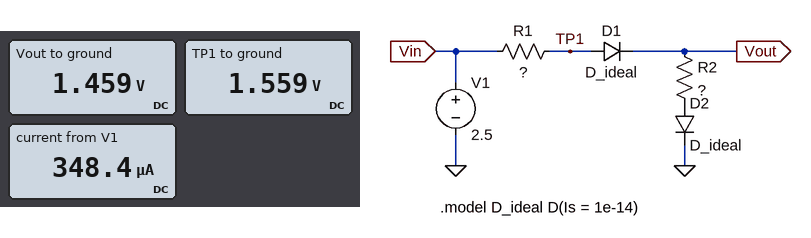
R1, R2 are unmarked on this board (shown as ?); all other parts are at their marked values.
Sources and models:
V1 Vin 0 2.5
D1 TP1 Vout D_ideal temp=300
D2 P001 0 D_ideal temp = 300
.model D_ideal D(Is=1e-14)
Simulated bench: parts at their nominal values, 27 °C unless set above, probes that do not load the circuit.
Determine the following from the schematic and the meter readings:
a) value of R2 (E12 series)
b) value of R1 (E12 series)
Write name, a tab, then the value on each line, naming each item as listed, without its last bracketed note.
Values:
value of R2	3.9 kΩ
value of R1	2.7 kΩ
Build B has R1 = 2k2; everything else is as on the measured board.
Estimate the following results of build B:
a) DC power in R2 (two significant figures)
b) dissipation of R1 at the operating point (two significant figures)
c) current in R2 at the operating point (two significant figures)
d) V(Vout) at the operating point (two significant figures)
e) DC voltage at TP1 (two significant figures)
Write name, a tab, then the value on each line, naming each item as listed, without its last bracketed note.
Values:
DC power in R2	550 µW
dissipation of R1 at the operating point	310 µW
current in R2 at the operating point	380 µA
V(Vout) at the operating point	1.6 V
DC voltage at TP1	1.7 V
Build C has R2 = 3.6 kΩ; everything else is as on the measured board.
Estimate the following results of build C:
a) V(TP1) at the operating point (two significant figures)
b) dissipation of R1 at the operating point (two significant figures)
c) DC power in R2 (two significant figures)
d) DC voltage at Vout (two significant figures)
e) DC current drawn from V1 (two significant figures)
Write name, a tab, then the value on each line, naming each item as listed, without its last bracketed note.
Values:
V(TP1) at the operating point	1.5 V
dissipation of R1 at the operating point	360 µW
DC power in R2	480 µW
DC voltage at Vout	1.4 V
DC current drawn from V1	360 µA
